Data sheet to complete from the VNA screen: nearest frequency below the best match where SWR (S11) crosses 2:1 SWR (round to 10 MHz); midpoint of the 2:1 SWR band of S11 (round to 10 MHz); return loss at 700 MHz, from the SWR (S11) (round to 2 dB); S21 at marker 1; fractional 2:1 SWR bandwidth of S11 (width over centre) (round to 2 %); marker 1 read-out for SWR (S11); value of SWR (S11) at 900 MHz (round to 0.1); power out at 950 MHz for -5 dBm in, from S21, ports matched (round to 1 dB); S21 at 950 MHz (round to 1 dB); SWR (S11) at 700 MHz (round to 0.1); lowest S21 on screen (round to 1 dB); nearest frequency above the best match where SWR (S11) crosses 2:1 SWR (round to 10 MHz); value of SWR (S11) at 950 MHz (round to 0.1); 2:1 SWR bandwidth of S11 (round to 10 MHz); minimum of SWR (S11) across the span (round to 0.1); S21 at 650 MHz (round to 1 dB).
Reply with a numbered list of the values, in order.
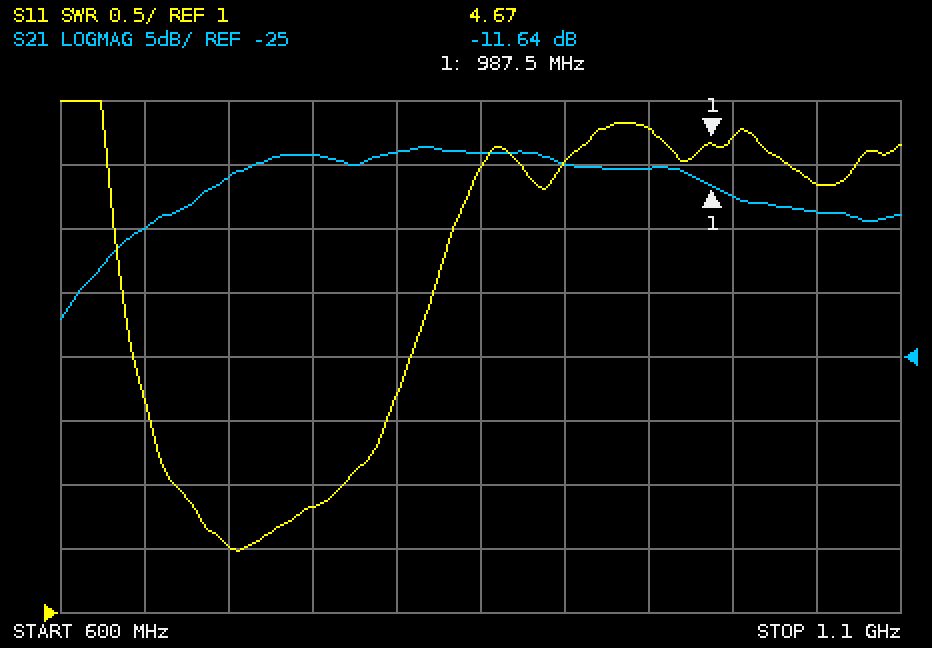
1. 670 MHz
2. 720 MHz
3. 14 dB
4. -11.64 dB
5. 14 %
6. 4.67
7. 4.5
8. -15 dBm
9. -10 dB
10. 1.5
11. -22 dB
12. 770 MHz
13. 4.8
14. 100 MHz
15. 1.5
16. -15 dB
